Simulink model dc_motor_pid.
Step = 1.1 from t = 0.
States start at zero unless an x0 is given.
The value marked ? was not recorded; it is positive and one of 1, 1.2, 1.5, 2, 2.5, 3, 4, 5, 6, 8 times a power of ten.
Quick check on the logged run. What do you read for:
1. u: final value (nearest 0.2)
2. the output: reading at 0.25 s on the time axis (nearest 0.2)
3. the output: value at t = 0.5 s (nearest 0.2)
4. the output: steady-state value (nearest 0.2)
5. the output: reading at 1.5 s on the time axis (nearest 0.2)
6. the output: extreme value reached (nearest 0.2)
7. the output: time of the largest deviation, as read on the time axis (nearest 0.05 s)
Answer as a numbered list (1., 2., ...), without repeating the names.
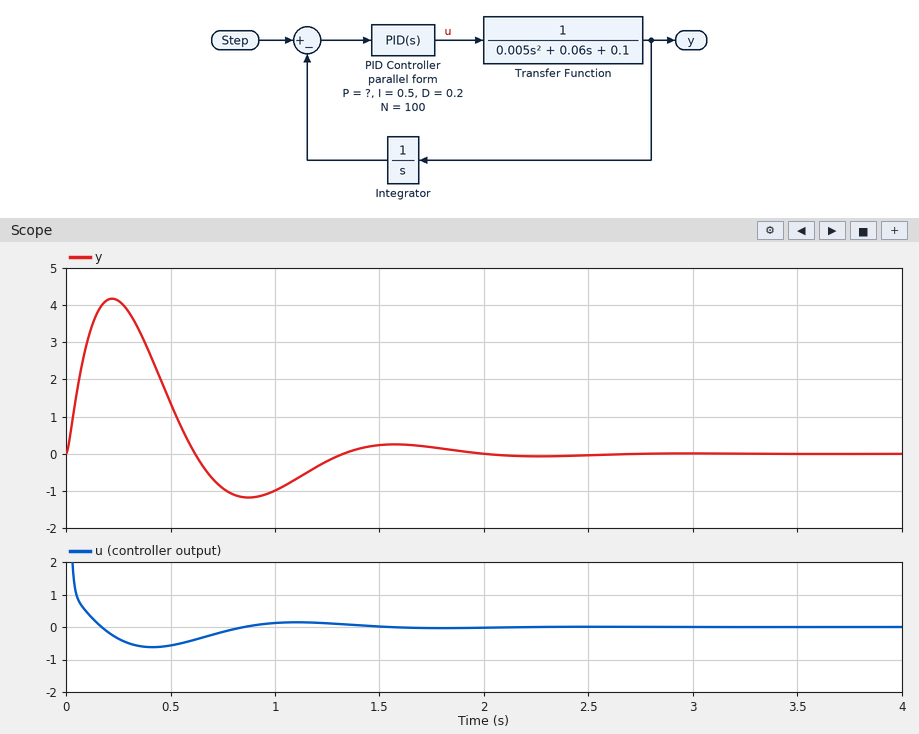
1. 0.0
2. 4.2
3. 1.4
4. 0.0
5. 0.2
6. 4.2
7. 0.20 s
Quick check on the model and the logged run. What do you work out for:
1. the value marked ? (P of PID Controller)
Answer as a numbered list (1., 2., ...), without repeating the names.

1. 1
